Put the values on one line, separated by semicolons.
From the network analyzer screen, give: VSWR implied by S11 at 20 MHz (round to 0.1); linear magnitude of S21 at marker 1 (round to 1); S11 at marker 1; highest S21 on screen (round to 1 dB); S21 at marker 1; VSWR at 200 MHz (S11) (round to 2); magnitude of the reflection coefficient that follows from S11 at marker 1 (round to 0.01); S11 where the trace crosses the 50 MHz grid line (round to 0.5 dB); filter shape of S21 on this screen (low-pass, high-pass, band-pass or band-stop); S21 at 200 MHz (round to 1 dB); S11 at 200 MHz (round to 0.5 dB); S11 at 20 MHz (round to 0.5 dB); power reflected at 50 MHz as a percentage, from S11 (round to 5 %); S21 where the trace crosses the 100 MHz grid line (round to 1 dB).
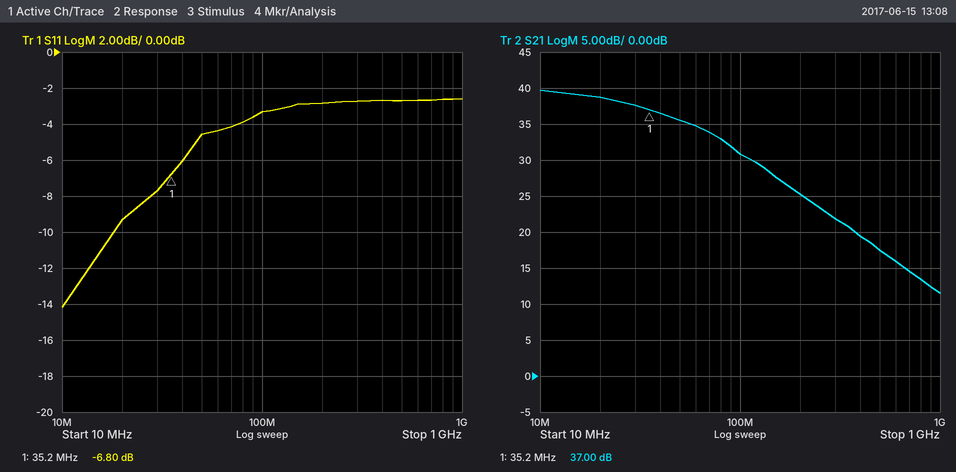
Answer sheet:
2.0; 71; -6.80 dB; 40 dB; 37.00 dB; 6; 0.46; -4.5 dB; low-pass; 25 dB; -3.0 dB; -9.5 dB; 35 %; 31 dB
